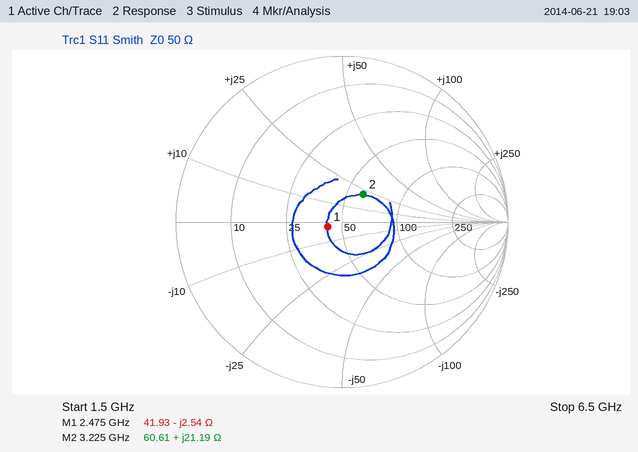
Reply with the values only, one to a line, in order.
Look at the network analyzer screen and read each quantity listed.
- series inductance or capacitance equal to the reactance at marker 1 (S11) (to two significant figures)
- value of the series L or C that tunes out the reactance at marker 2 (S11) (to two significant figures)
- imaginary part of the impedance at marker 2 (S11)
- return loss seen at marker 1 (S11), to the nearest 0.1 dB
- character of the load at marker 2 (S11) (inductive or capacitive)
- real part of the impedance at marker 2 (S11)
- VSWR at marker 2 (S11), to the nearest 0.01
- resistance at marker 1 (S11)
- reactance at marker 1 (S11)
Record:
25 pF
2.3 pF
+21.19 Ω
20.7 dB
inductive
60.61 Ω
1.53
41.93 Ω
-2.54 Ω
